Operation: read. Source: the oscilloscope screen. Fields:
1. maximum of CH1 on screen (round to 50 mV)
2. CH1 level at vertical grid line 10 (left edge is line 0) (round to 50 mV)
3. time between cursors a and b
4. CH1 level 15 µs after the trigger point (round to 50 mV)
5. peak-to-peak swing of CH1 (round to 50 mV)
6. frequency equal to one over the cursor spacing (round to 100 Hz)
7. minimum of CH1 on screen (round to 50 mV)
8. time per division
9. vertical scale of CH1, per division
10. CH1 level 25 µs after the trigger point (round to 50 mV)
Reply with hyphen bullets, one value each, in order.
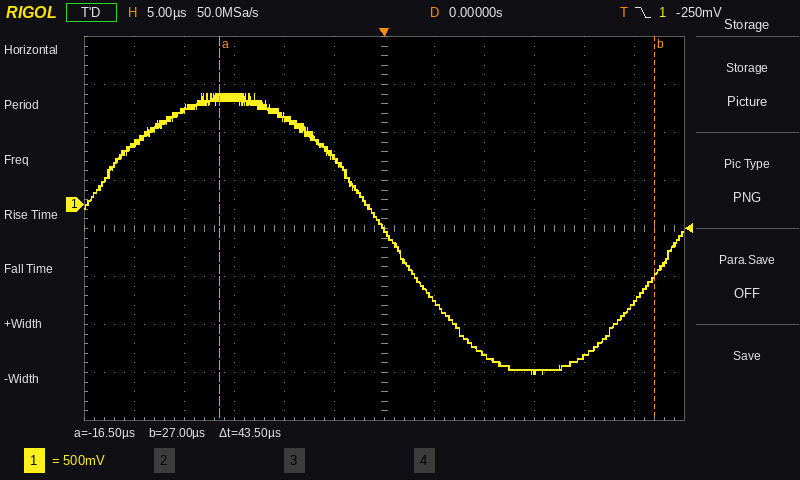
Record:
- 1.15 V
- -1.60 V
- 43.5 µs
- -1.75 V
- 2.90 V
- 23.0 kHz
- -1.75 V
- 5 µs
- 500 mV
- -1.00 V
